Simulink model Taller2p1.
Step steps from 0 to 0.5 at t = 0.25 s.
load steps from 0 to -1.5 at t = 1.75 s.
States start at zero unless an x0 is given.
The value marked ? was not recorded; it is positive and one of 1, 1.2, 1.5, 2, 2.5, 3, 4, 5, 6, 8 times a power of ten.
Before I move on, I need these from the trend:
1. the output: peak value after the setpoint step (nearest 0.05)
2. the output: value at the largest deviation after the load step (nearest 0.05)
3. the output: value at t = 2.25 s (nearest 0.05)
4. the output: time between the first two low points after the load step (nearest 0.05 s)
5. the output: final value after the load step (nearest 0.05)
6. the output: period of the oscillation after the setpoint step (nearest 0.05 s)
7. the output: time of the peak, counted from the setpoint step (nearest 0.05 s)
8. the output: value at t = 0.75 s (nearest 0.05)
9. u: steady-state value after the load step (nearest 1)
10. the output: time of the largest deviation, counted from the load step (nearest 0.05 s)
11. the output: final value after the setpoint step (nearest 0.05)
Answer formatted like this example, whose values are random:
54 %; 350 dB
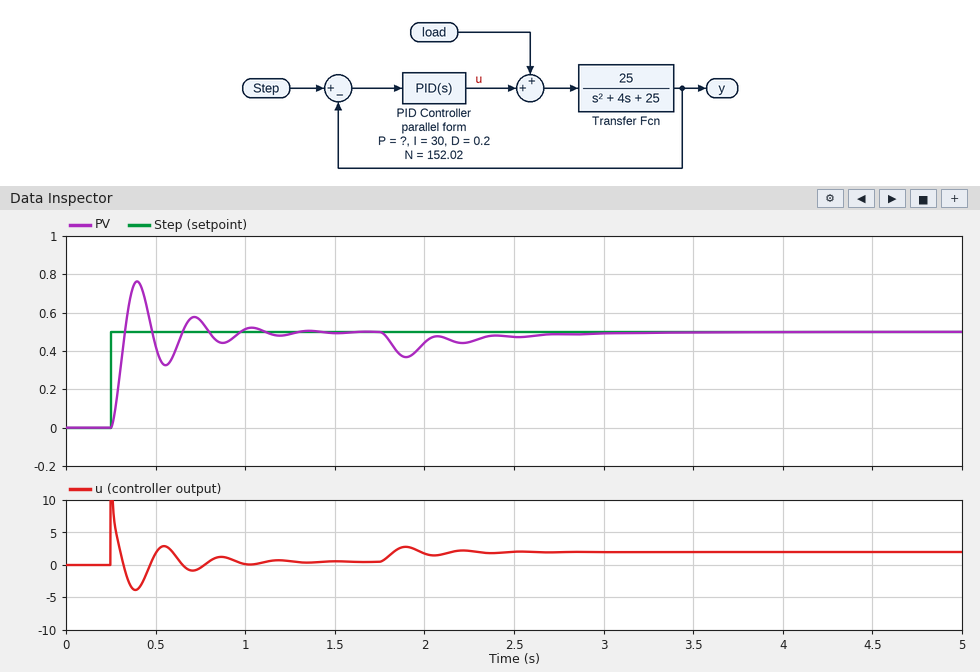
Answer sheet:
0.75; 0.35; 0.45; 0.30 s; 0.50; 0.30 s; 0.15 s; 0.55; 2; 0.15 s; 0.50
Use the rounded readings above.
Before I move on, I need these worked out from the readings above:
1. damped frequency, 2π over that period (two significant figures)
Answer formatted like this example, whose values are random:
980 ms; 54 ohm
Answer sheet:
21 rad/s
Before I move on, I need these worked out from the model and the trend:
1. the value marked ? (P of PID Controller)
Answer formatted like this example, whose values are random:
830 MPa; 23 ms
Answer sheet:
15
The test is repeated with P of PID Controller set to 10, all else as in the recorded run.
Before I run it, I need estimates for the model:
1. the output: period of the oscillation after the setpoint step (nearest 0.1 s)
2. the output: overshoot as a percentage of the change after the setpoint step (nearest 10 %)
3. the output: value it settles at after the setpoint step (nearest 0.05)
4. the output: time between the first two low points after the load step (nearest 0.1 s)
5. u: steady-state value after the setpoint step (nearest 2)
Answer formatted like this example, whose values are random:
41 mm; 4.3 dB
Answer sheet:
0.4 s; 50 %; 0.50; 0.4 s; 0
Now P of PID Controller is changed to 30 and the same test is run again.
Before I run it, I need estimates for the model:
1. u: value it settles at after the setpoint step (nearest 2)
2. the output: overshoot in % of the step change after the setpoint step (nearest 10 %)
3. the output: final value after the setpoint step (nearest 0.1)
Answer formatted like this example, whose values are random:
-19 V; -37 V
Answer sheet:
0; 60 %; 0.5
